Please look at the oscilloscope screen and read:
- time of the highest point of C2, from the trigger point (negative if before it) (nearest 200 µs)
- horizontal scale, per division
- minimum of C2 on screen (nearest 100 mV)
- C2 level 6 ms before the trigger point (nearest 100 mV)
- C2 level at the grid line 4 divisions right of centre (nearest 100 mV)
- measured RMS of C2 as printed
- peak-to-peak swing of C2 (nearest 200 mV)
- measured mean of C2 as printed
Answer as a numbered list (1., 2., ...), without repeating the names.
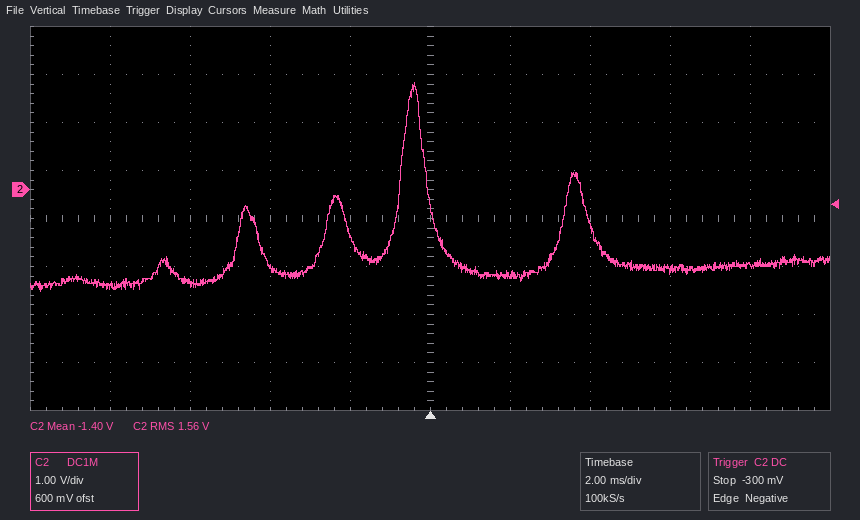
1. -400 µs
2. 2 ms
3. -2.1 V
4. -1.9 V
5. -1.6 V
6. 1.56 V
7. 4.4 V
8. -1.40 V
